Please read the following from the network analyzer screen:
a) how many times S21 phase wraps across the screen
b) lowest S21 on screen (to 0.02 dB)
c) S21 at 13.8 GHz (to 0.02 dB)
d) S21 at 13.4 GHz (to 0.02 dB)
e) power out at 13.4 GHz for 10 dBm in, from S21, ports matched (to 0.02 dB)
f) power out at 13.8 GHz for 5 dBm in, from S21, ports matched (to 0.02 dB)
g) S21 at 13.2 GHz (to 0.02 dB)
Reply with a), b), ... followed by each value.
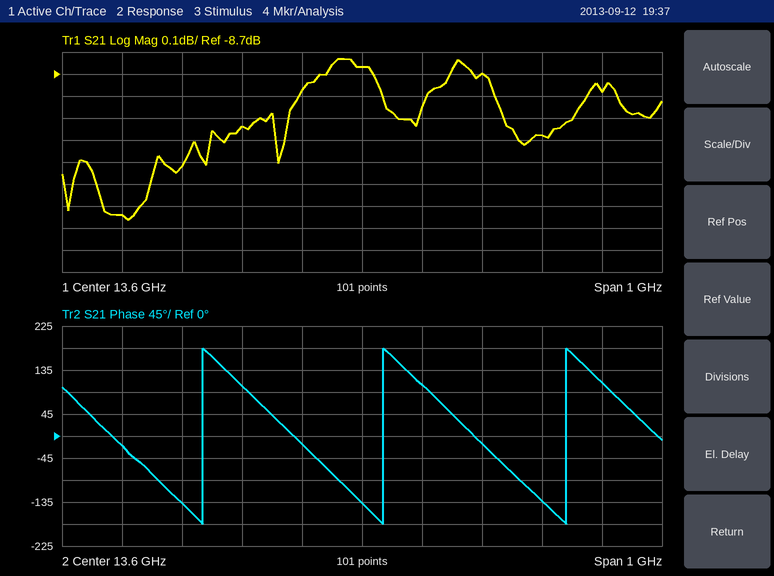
a) 3
b) -9.36 dB
c) -8.70 dB
d) -8.94 dB
e) 1.06 dBm
f) -3.70 dBm
g) -9.34 dB
